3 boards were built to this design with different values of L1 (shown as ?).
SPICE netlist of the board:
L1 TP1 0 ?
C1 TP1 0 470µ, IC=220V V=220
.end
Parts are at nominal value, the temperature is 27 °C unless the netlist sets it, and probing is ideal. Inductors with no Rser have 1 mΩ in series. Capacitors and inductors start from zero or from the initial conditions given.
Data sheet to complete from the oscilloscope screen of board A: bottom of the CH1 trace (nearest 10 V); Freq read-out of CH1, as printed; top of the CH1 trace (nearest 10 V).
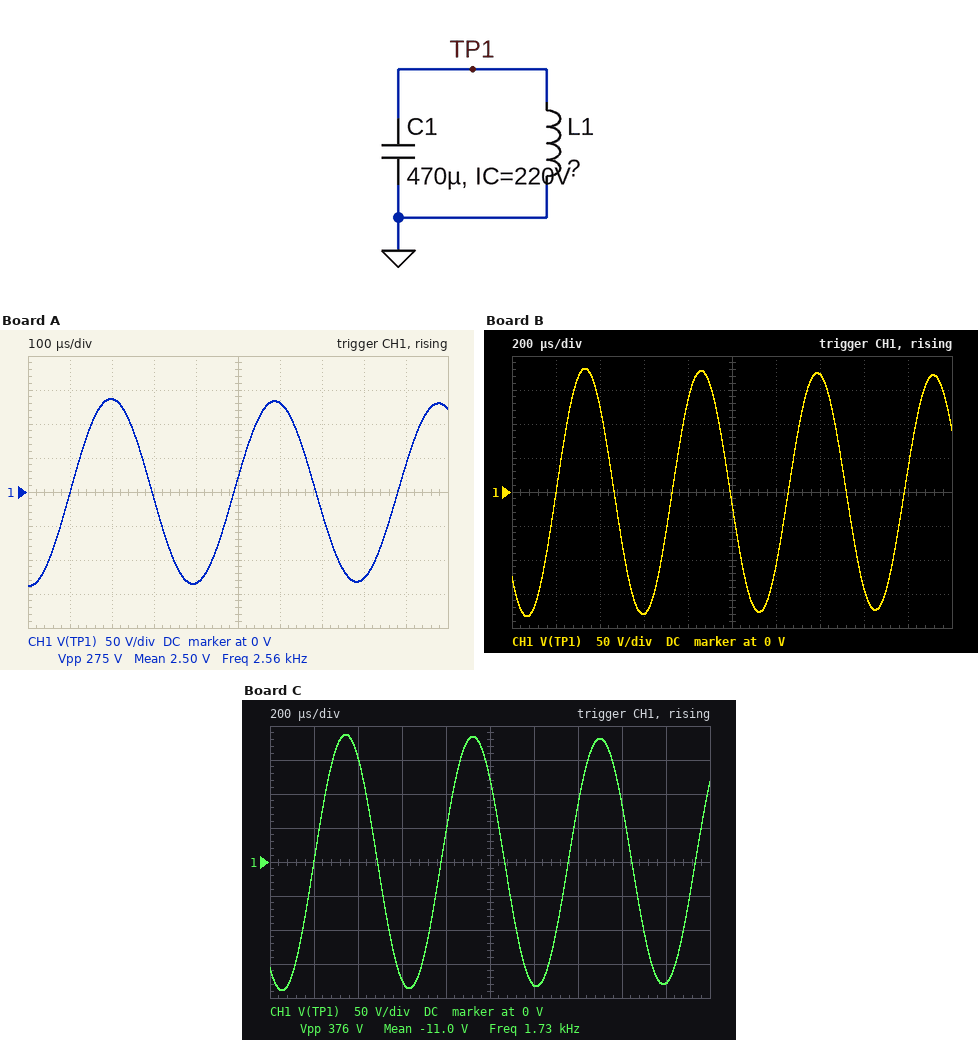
-140 V
2.56 kHz
140 V
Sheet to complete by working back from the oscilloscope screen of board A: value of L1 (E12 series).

8.2 µH
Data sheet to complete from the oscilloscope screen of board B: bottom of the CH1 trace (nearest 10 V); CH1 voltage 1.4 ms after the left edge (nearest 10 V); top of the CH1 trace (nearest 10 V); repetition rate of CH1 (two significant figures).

-180 V
170 V
180 V
1.9 kHz
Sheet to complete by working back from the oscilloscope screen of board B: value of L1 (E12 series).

15 µH
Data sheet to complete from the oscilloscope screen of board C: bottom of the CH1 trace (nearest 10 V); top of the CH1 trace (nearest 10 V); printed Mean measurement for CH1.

-190 V
190 V
-11.0 V
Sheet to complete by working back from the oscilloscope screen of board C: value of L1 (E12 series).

18 µH
